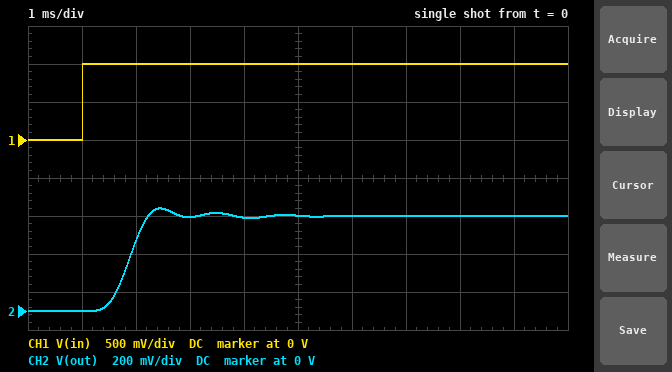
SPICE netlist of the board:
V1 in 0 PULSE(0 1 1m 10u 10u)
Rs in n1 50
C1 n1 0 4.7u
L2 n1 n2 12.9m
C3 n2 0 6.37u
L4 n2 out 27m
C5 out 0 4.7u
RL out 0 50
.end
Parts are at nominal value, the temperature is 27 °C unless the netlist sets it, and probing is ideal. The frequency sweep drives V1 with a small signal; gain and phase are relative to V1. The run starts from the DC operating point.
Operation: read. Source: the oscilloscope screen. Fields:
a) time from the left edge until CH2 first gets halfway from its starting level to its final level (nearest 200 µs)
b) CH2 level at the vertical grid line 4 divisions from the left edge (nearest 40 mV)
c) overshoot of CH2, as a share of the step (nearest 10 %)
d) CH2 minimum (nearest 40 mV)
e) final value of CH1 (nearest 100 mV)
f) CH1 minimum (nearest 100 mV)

1.8 ms
480 mV
10 %
0 V
1.0 V
0 V
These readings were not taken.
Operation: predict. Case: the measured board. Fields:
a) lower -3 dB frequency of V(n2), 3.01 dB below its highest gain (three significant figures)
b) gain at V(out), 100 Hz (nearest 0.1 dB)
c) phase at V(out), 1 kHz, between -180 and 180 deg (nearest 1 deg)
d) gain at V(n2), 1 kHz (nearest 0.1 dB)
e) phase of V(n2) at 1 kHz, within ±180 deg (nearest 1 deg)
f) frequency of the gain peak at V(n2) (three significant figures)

610 Hz
-6.0 dB
16 deg
-5.6 dB
156 deg
804 Hz
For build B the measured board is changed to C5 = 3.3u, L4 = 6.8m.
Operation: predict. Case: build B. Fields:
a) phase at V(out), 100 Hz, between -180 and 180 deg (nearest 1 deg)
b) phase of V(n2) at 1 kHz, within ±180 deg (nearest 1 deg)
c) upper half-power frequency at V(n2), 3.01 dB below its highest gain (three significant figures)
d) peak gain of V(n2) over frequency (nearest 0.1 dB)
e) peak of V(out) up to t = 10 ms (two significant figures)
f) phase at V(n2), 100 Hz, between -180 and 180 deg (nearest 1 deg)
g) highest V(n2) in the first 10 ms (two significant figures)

-20 deg
-138 deg
790 Hz
-6.0 dB
550 mV
-15 deg
500 mV
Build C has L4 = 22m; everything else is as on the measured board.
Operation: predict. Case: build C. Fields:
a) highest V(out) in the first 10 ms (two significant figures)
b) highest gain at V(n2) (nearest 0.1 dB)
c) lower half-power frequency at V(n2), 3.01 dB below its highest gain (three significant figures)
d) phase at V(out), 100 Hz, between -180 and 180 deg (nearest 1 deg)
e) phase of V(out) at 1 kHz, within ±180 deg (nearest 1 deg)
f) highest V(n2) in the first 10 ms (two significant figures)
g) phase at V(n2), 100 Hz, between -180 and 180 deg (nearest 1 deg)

560 mV
1.1 dB
660 Hz
-27 deg
21 deg
680 mV
-11 deg
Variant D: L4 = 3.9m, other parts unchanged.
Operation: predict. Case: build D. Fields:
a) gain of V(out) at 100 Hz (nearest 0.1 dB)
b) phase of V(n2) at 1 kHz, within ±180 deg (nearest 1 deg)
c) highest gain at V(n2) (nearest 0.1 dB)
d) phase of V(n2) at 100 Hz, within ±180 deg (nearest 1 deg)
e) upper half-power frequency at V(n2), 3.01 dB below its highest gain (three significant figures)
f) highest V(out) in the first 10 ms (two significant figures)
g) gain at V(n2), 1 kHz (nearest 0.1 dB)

-6.1 dB
-146 deg
-6.0 dB
-17 deg
629 Hz
520 mV
-17.5 dB
